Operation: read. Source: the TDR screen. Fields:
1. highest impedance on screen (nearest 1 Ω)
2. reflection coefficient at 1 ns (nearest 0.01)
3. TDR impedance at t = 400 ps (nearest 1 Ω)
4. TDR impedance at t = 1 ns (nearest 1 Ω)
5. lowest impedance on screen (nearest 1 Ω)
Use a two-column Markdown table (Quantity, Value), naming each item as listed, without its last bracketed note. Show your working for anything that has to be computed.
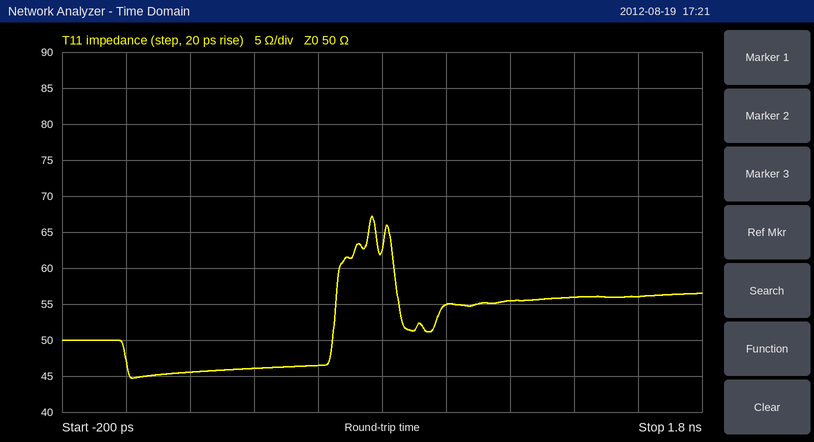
| Quantity | Value |
|---|---|
| highest impedance on screen | 67 Ω |
| reflection coefficient at 1 ns | (55 − 50)/(55 + 50) ≈ +0.05 |
| TDR impedance at t = 400 ps | 46 Ω |
| TDR impedance at t = 1 ns | 55 Ω |
| lowest impedance on screen | 45 Ω |
